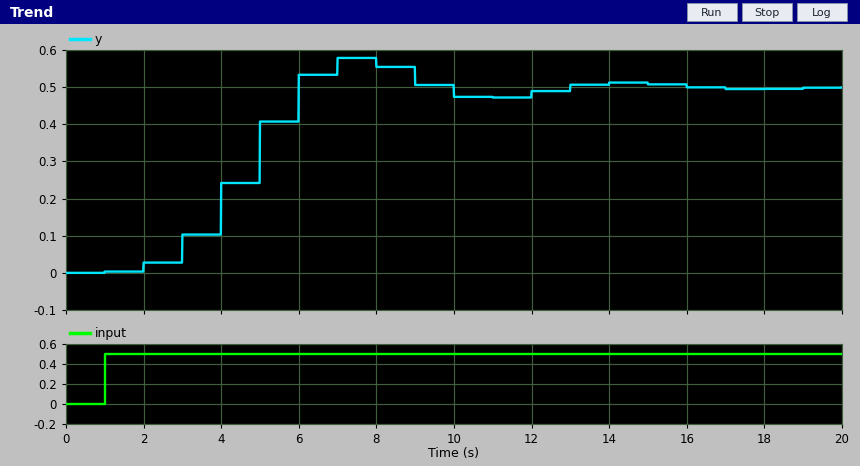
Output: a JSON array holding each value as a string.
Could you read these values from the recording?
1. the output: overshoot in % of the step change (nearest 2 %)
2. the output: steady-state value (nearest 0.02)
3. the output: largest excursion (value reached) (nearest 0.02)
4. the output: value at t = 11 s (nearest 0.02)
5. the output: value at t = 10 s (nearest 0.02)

["16 %", "0.50", "0.58", "0.48", "0.48"]
